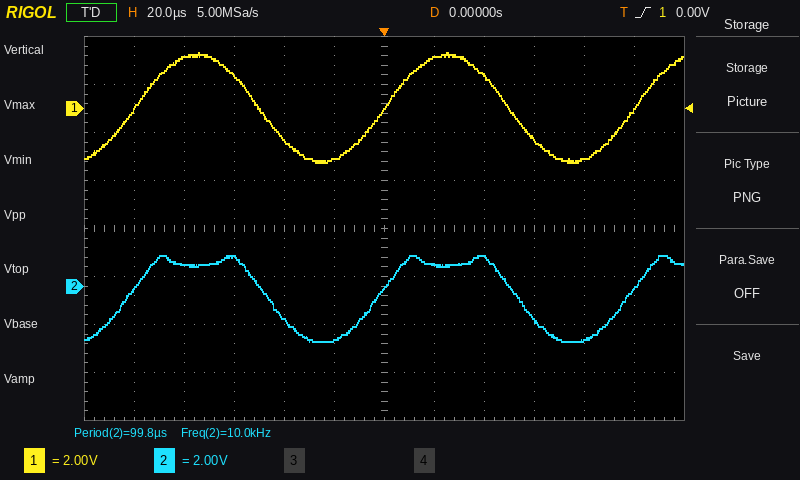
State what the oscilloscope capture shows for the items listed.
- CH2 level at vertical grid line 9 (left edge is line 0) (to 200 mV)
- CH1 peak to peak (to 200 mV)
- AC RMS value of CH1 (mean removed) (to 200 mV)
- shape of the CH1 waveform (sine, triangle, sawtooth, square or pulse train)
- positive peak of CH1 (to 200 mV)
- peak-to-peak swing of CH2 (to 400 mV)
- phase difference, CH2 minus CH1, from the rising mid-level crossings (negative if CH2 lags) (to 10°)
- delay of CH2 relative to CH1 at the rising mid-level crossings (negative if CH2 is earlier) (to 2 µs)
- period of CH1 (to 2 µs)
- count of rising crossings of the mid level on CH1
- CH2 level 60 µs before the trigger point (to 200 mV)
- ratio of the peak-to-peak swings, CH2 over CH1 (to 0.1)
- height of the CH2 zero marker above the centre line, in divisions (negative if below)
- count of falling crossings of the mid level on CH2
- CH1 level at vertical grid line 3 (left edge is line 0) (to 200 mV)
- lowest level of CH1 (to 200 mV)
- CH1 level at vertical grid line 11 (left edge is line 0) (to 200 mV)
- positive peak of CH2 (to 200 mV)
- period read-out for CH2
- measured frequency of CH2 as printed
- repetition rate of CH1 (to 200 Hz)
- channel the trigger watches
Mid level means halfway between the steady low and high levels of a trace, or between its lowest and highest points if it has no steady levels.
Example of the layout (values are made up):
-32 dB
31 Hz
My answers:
-1.4 V
4.6 V
1.6 V
sine
2.4 V
3.6 V
+10°
-4 µs
100 µs
3
1.2 V
0.8
-1.2 div
2
1.4 V
-2.2 V
0.0 V
1.2 V
99.8 µs
10.0 kHz
10.0 kHz
CH1
